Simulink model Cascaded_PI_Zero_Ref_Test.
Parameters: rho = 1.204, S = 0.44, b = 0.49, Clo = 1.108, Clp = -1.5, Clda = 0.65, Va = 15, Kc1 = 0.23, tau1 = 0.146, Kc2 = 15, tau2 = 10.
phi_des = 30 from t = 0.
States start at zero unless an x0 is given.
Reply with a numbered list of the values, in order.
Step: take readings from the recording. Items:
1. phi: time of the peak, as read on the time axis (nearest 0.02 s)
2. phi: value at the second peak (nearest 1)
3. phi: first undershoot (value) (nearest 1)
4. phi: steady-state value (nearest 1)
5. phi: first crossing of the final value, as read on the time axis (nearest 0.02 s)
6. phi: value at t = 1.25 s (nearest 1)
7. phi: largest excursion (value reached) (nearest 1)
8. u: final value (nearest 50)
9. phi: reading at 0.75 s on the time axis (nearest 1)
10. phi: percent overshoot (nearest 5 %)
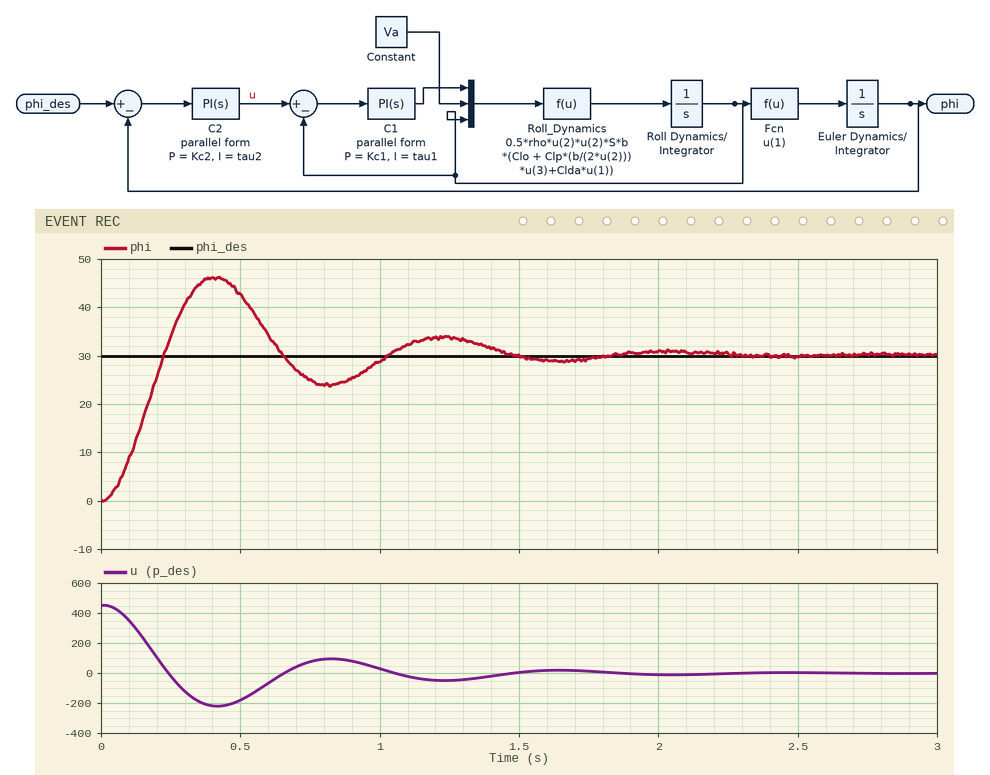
1. 0.40 s
2. 34
3. 24
4. 30
5. 0.22 s
6. 34
7. 46
8. 0
9. 25
10. 55 %
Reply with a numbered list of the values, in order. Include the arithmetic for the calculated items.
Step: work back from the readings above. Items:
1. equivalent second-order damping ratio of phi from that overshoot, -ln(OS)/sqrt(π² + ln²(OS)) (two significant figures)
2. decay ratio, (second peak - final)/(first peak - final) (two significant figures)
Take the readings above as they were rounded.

1. ln(0.55) = -0.598; 0.598 / sqrt(9.870 + 0.357) = 0.19
2. (34 - 30) / (46 - 30) = 0.25
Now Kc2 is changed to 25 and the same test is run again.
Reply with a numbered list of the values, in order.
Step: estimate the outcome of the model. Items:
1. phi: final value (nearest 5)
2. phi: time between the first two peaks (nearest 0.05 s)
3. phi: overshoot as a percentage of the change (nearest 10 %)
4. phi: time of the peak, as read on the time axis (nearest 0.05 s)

1. 30
2. 0.60 s
3. 60 %
4. 0.30 s
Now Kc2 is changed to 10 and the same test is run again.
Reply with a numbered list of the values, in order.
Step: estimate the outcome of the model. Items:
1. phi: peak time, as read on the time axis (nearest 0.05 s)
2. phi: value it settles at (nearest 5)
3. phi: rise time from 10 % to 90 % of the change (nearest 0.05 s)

1. 0.50 s
2. 30
3. 0.20 s
